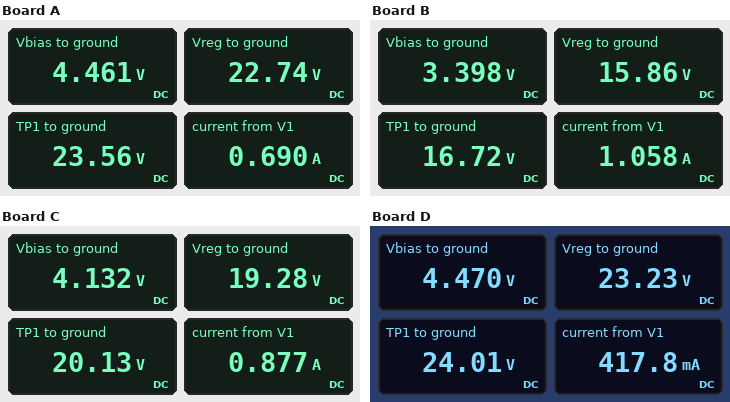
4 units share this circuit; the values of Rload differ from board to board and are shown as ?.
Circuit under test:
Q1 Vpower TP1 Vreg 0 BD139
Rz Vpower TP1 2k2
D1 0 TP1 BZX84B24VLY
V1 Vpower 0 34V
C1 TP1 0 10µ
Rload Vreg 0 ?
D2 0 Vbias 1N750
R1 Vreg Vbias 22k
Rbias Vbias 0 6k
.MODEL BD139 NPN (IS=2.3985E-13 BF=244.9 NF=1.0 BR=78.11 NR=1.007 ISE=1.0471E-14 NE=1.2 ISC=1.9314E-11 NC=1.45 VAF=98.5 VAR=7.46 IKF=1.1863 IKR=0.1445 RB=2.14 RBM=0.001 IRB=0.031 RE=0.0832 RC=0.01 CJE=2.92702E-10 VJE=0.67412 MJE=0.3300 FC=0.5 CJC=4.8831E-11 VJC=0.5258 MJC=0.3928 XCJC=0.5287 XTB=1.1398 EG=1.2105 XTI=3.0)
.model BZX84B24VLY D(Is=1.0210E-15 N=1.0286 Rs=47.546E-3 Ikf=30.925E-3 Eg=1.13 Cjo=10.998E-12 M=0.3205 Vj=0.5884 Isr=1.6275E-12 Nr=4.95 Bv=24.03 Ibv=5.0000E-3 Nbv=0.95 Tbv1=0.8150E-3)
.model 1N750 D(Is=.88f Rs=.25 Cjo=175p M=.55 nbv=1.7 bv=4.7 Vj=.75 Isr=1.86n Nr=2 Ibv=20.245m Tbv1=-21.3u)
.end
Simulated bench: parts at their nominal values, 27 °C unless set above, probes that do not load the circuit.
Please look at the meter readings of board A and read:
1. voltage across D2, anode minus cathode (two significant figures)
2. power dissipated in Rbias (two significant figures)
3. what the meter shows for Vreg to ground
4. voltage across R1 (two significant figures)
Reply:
-4.5 V
3.3 mW
22.74 V
18 V
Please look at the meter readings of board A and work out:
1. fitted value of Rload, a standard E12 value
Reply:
33 Ω
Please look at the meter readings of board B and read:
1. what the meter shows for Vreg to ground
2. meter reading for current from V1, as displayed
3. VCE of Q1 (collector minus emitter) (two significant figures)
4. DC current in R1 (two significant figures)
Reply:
15.86 V
1.058 A
18 V
570 µA
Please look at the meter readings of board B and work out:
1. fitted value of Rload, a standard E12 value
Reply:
15 Ω
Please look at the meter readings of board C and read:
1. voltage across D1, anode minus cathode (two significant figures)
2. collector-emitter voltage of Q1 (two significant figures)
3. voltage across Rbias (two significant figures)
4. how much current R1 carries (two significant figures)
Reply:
-20 V
15 V
4.1 V
690 µA
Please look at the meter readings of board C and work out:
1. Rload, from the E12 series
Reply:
22 Ω
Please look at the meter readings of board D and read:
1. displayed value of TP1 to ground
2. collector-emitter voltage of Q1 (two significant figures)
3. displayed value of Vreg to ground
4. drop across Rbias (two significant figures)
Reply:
24.01 V
11 V
23.23 V
4.5 V
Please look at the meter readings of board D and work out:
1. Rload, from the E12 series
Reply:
56 Ω
